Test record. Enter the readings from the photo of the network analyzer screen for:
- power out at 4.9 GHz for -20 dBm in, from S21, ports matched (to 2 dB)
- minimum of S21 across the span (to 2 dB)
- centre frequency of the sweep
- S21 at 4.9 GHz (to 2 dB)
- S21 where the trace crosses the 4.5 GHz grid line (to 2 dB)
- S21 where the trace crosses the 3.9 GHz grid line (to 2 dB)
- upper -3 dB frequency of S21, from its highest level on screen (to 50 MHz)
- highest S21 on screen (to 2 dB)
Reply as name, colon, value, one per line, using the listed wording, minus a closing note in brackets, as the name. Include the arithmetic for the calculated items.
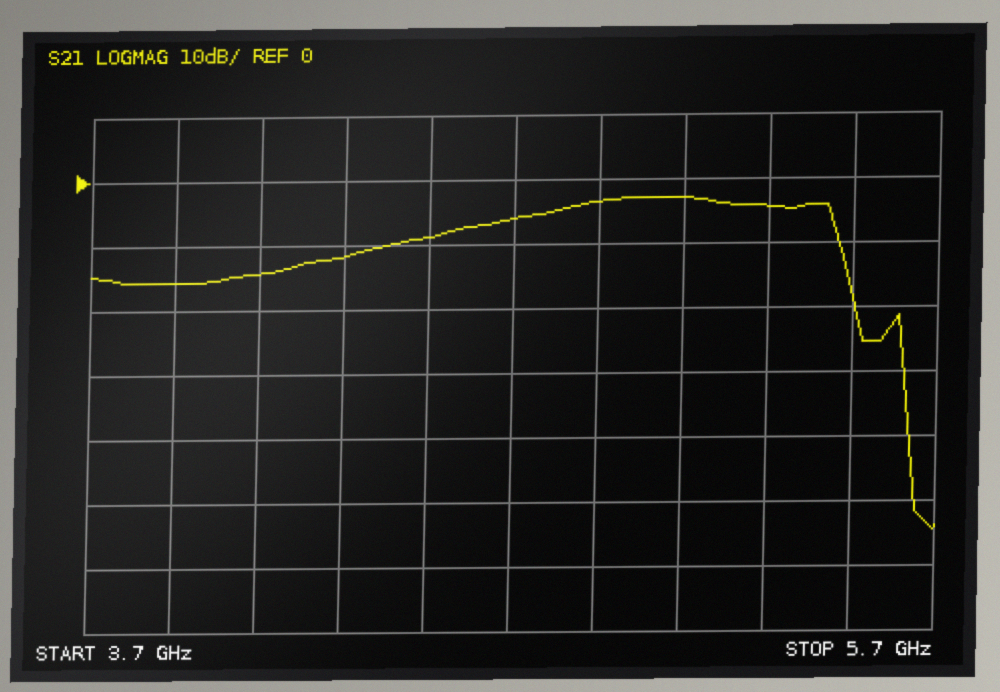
power out at 4.9 GHz for -20 dBm in, from S21, ports matched: -20 dBm + (-4 dB) = -24 dBm
minimum of S21 across the span: -54 dB
centre frequency of the sweep: 4.7 GHz
S21 at 4.9 GHz: -4 dB
S21 where the trace crosses the 4.5 GHz grid line: -8 dB
S21 where the trace crosses the 3.9 GHz grid line: -16 dB
upper -3 dB frequency of S21, from its highest level on screen: 5.45 GHz
highest S21 on screen: -2 dB
